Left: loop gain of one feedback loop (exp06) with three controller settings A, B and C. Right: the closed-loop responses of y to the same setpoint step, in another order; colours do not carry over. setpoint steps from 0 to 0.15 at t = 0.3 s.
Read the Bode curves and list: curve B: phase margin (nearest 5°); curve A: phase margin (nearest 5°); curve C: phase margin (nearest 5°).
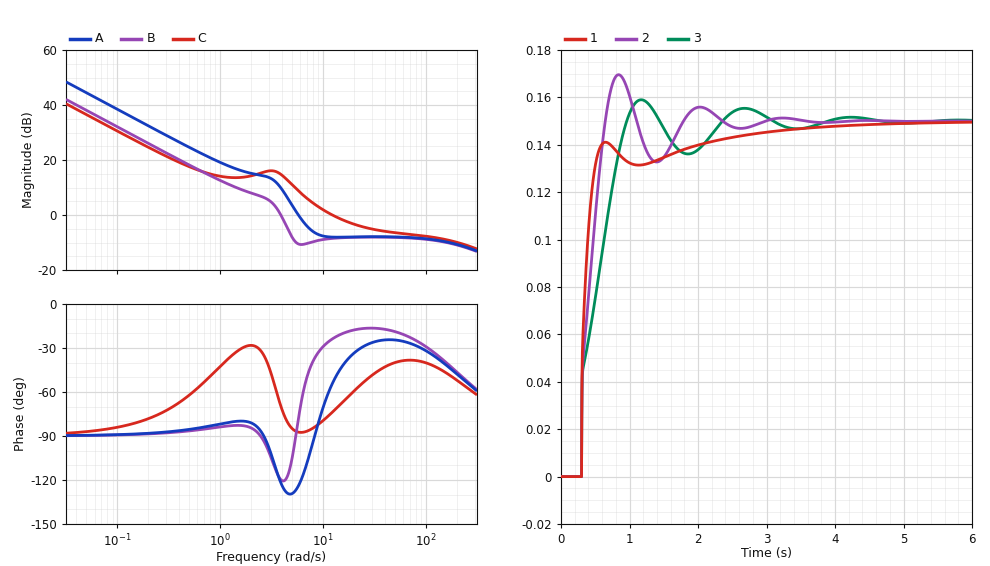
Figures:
60°
55°
105°
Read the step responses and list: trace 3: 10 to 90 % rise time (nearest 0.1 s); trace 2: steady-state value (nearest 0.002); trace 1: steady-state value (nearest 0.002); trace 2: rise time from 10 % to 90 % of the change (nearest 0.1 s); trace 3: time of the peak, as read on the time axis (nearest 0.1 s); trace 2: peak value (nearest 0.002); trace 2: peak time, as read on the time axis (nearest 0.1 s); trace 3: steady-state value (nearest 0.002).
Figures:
0.5 s
0.150
0.150
0.3 s
1.2 s
0.170
0.8 s
0.150
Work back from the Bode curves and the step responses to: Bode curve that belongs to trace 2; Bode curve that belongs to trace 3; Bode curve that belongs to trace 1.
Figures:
A
B
C
